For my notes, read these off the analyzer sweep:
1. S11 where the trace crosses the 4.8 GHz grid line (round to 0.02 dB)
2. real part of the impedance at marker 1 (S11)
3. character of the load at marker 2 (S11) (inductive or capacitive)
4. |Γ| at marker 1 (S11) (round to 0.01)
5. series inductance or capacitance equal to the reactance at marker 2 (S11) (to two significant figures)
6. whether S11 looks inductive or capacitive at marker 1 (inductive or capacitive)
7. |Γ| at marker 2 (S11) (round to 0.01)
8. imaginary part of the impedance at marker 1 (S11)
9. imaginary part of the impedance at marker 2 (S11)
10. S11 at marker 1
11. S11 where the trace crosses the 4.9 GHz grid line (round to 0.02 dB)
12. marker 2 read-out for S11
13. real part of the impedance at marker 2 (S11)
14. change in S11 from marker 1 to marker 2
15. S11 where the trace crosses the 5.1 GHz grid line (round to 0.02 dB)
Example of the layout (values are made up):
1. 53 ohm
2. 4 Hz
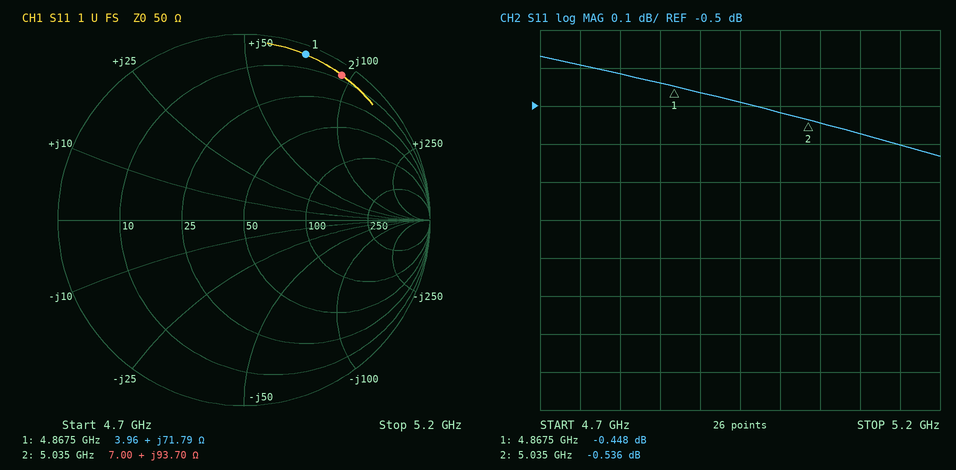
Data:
1. -0.42 dB
2. 3.96 Ω
3. inductive
4. 0.95
5. 3.0 nH
6. inductive
7. 0.94
8. +71.79 Ω
9. +93.70 Ω
10. -0.448 dB
11. -0.46 dB
12. -0.536 dB
13. 7.00 Ω
14. -0.088 dB
15. -0.58 dB
